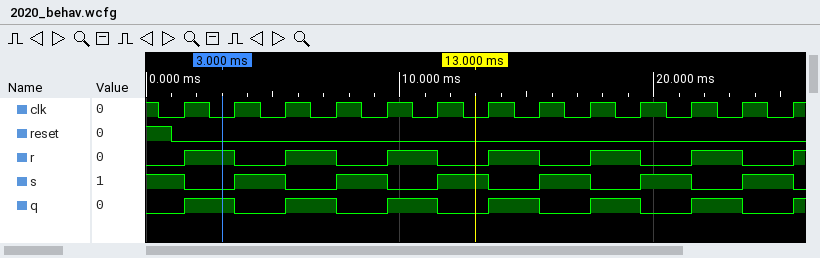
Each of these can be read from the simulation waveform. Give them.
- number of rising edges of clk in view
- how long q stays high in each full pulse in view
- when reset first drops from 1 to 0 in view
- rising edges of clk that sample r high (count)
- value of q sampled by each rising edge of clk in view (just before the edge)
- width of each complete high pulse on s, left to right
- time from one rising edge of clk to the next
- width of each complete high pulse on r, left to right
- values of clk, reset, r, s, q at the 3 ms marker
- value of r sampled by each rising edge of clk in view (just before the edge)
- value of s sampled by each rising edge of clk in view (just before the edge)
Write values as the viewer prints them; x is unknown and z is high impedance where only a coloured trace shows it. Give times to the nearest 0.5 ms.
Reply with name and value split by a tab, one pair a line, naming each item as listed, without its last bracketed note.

number of rising edges of clk in view	13
how long q stays high in each full pulse in view	2 ms, 2 ms, 2 ms, 2 ms, 2 ms, 2 ms
when reset first drops from 1 to 0 in view	1 ms
rising edges of clk that sample r high	6
value of q sampled by each rising edge of clk in view	0 1 0 1 0 1 0 1 0 1 0 1 0
width of each complete high pulse on s, left to right	2 ms, 2 ms, 2 ms, 2 ms, 2 ms, 2 ms
time from one rising edge of clk to the next	2 ms
width of each complete high pulse on r, left to right	2 ms, 2 ms, 2 ms, 2 ms, 2 ms, 2 ms
values of clk, reset, r, s, q at the 3 ms marker	clk=0, reset=0, r=1, s=0, q=1
value of r sampled by each rising edge of clk in view	0 1 0 1 0 1 0 1 0 1 0 1 0
value of s sampled by each rising edge of clk in view	1 0 1 0 1 0 1 0 1 0 1 0 1
